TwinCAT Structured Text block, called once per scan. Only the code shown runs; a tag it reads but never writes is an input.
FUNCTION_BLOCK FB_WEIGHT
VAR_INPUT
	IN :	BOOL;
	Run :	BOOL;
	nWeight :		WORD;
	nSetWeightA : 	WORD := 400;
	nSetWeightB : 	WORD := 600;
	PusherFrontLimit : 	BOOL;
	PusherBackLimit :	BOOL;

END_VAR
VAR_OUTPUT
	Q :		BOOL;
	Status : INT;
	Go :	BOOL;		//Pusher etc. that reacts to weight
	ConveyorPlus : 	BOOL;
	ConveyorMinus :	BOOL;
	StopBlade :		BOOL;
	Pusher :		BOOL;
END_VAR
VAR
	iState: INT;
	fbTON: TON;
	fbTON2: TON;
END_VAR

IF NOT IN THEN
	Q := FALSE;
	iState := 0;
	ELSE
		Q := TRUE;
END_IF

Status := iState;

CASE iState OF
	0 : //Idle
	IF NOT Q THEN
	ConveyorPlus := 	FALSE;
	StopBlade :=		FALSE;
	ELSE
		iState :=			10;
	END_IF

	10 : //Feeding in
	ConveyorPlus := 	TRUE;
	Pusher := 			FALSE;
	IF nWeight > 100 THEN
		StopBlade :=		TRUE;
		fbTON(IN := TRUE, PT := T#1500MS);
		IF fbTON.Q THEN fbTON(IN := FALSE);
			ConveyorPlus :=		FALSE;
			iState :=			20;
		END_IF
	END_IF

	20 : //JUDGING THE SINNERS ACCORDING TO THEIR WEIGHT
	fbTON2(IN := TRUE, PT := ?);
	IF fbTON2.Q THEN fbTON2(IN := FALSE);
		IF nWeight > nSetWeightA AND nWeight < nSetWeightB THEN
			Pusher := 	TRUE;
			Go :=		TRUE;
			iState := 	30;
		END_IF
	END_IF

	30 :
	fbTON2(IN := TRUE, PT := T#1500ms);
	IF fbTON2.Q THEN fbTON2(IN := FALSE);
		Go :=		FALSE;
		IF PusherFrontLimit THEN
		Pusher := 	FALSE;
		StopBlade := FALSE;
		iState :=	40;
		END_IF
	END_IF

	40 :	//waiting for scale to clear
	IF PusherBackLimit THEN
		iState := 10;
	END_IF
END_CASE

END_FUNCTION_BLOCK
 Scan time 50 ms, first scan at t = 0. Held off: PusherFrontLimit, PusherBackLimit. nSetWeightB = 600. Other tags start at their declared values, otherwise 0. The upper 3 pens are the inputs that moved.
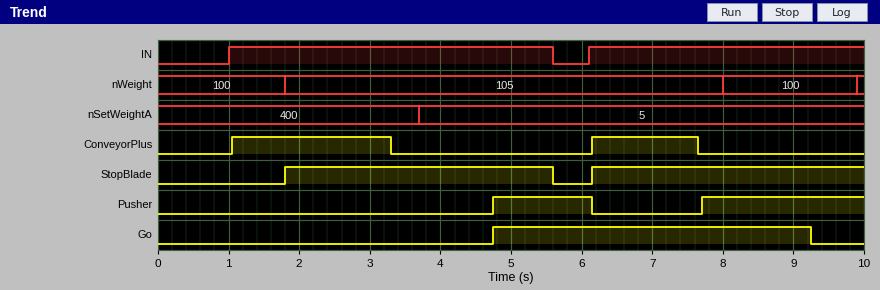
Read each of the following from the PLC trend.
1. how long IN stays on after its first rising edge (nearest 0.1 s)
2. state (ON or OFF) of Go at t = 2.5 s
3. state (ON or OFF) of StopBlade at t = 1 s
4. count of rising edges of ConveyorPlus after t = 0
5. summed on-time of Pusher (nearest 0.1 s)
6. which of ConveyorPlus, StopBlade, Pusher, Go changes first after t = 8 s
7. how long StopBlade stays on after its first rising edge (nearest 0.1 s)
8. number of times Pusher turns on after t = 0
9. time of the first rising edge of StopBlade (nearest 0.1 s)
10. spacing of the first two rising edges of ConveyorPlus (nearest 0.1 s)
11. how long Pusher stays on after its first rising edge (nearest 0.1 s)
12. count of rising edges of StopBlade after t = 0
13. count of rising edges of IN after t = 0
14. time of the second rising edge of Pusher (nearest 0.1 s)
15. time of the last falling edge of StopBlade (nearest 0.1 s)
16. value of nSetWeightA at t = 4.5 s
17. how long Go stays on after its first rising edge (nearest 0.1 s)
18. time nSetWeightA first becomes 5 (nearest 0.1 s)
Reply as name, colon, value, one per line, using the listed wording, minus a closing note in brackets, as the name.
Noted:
how long IN stays on after its first rising edge: 4.6 s
state (ON or OFF) of Go at t = 2.5 s: OFF
state (ON or OFF) of StopBlade at t = 1 s: OFF
count of rising edges of ConveyorPlus after t = 0: 2
summed on-time of Pusher: 3.7 s
which of ConveyorPlus, StopBlade, Pusher, Go changes first after t = 8 s: Go
how long StopBlade stays on after its first rising edge: 3.8 s
number of times Pusher turns on after t = 0: 2
time of the first rising edge of StopBlade: 1.8 s
spacing of the first two rising edges of ConveyorPlus: 5.1 s
how long Pusher stays on after its first rising edge: 1.4 s
count of rising edges of StopBlade after t = 0: 2
count of rising edges of IN after t = 0: 2
time of the second rising edge of Pusher: 7.7 s
time of the last falling edge of StopBlade: 5.6 s
value of nSetWeightA at t = 4.5 s: 5
how long Go stays on after its first rising edge: 4.5 s
time nSetWeightA first becomes 5: 3.7 s
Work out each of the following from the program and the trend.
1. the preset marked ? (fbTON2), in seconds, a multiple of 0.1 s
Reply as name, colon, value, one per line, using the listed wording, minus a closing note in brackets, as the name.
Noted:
the preset marked ? (fbTON2), in seconds, a multiple of 0.1 s: 1.4 s
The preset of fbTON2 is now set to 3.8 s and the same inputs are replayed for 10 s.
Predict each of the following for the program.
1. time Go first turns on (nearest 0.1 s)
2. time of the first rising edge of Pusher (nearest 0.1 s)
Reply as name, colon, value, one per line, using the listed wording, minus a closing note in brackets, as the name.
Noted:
time Go first turns on: 7.7 s
time of the first rising edge of Pusher: 7.7 s
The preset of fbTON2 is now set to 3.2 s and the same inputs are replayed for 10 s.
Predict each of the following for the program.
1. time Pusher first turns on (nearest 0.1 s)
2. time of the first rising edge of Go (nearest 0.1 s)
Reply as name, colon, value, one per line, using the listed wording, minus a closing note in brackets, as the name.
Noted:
time Pusher first turns on: 7.7 s
time of the first rising edge of Go: 7.7 s
